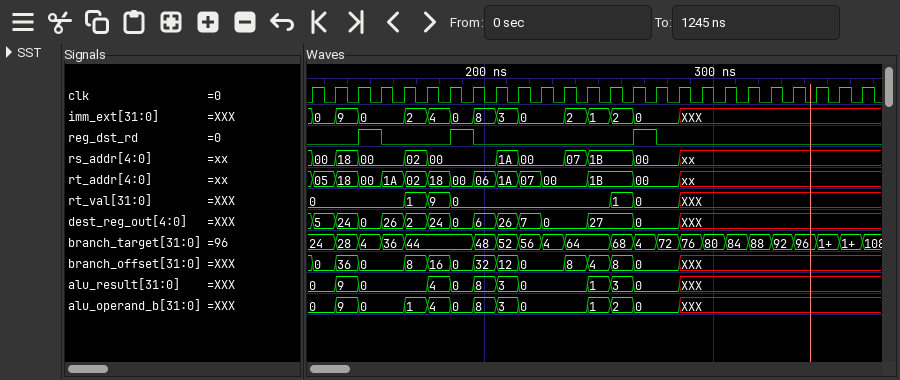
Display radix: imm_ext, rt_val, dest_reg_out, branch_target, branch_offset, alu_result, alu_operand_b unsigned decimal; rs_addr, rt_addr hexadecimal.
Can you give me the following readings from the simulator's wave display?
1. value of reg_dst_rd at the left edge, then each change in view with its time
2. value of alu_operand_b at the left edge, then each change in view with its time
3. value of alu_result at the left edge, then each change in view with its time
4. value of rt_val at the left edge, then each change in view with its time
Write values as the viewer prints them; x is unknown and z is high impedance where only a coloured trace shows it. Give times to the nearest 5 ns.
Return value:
0, 1 at 145 ns, 0 at 155 ns, 1 at 185 ns, 0 at 195 ns, 1 at 265 ns, 0 at 275 ns
0, 9 at 135 ns, 0 at 145 ns, 1 at 165 ns, 4 at 175 ns, 0 at 185 ns, 8 at 195 ns, 3 at 205 ns, 0 at 215 ns, 1 at 245 ns, 2 at 255 ns, 0 at 265 ns, XXX at 285 ns
0, 9 at 135 ns, 0 at 145 ns, 4 at 175 ns, 0 at 185 ns, 8 at 195 ns, 3 at 205 ns, 0 at 215 ns, 1 at 245 ns, 3 at 255 ns, 0 at 265 ns, XXX at 285 ns
0, 1 at 165 ns, 9 at 175 ns, 0 at 185 ns, 1 at 255 ns, 0 at 265 ns, XXX at 285 ns
